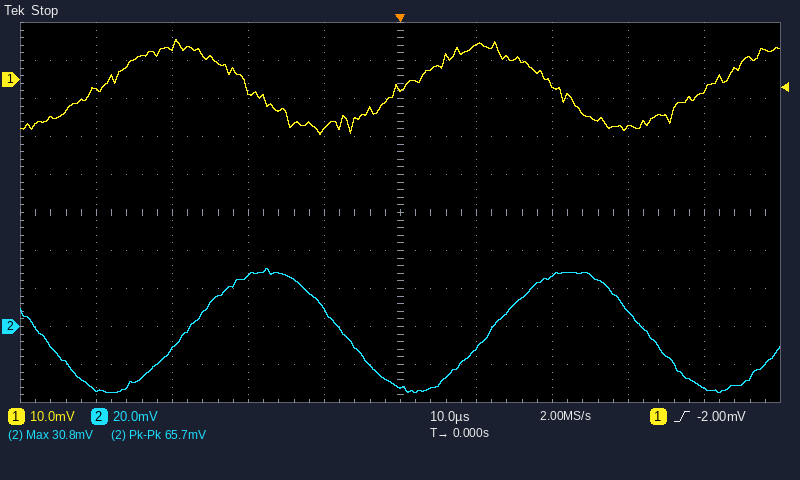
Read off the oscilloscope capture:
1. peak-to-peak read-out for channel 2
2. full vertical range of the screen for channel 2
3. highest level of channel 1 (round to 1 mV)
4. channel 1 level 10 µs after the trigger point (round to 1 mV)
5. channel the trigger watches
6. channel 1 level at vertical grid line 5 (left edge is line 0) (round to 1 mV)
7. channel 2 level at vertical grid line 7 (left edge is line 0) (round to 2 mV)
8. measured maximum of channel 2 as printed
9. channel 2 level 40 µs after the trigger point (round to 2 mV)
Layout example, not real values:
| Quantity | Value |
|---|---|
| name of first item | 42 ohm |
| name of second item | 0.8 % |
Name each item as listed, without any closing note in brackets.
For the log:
| Quantity | Value |
|---|---|
| peak-to-peak read-out for channel 2 | 65.7 mV |
| full vertical range of the screen for channel 2 | 200 mV |
| highest level of channel 1 | 11 mV |
| channel 1 level 10 µs after the trigger point | 9 mV |
| channel the trigger watches | channel 1 |
| channel 1 level at vertical grid line 5 (left edge is line 0) | -2 mV |
| channel 2 level at vertical grid line 7 (left edge is line 0) | 26 mV |
| measured maximum of channel 2 as printed | 30.8 mV |
| channel 2 level 40 µs after the trigger point | -32 mV |
